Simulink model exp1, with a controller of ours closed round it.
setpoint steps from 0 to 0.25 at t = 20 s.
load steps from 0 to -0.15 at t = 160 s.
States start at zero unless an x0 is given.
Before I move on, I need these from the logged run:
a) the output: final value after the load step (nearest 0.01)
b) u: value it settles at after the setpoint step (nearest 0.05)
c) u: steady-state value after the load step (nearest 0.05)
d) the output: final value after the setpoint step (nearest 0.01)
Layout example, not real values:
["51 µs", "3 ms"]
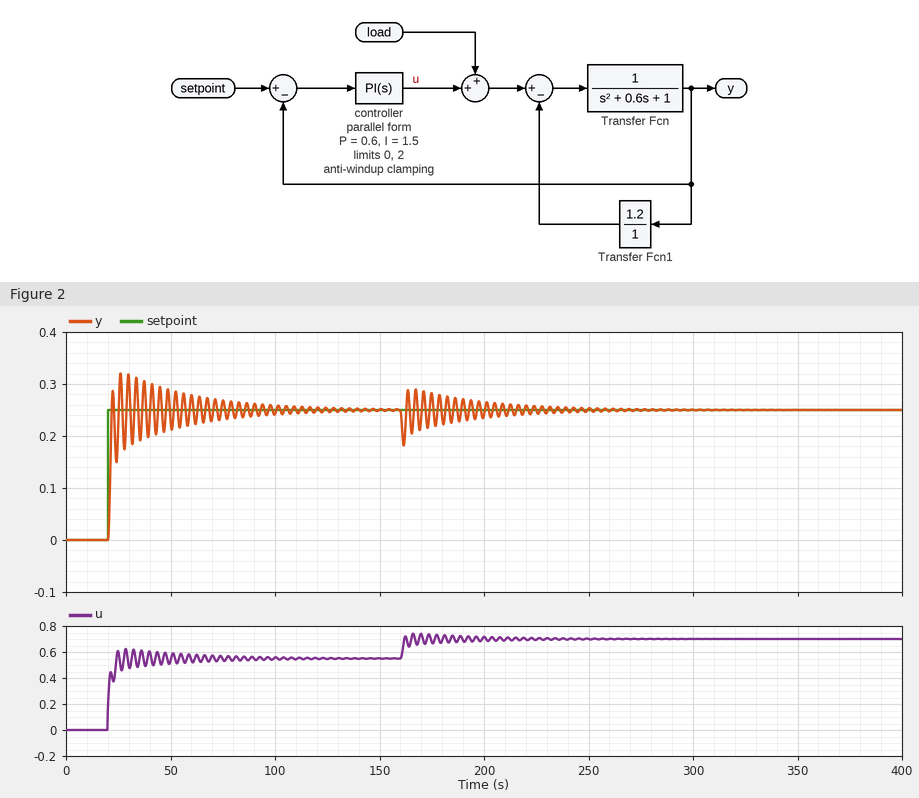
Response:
["0.25", "0.55", "0.70", "0.25"]
